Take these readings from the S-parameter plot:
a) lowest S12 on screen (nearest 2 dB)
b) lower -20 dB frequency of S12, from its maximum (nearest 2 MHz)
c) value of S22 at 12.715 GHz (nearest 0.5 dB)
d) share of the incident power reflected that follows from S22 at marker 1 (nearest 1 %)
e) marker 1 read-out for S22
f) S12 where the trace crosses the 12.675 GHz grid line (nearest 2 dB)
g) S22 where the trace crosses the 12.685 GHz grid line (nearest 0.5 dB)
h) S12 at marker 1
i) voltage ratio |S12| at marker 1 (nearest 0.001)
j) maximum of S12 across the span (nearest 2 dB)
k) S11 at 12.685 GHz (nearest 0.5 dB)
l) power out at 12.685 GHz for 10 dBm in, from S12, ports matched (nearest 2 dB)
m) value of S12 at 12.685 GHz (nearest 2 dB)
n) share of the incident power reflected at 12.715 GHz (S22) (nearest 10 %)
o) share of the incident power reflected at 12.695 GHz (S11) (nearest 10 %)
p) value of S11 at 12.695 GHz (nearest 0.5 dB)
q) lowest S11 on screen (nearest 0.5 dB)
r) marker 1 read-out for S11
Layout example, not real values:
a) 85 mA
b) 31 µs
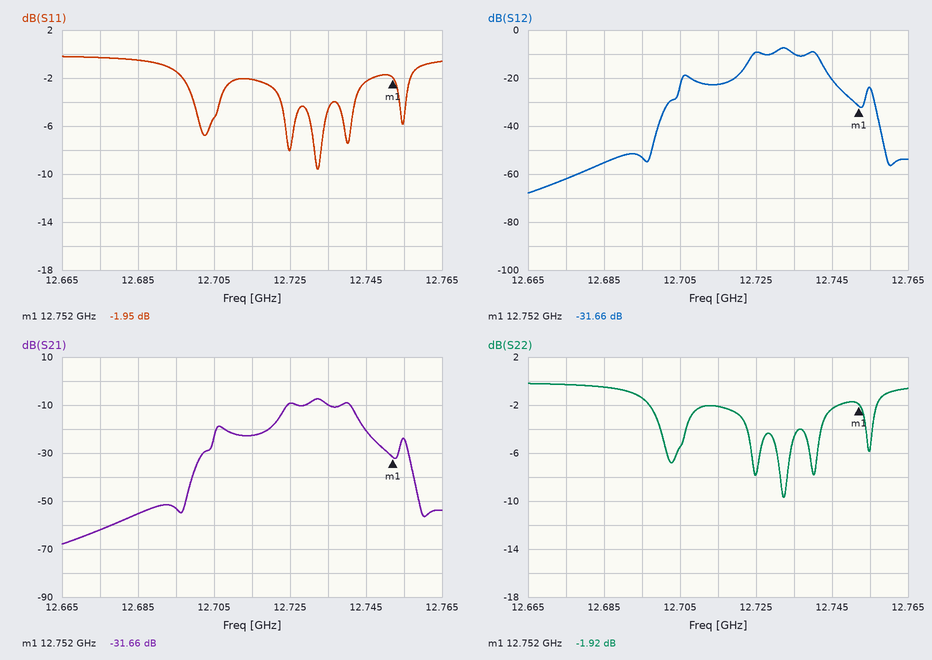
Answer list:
a) -68 dB
b) 12.704 GHz
c) -2.0 dB
d) 64 %
e) -1.92 dB
f) -62 dB
g) -0.5 dB
h) -31.66 dB
i) 0.026
j) -8 dB
k) -0.5 dB
l) -46 dBm
m) -56 dB
n) 60 %
o) 70 %
p) -1.5 dB
q) -9.5 dB
r) -1.95 dB
